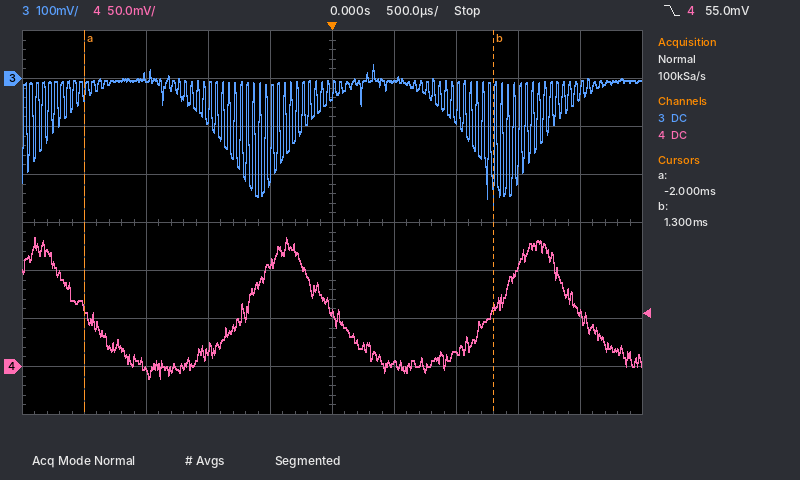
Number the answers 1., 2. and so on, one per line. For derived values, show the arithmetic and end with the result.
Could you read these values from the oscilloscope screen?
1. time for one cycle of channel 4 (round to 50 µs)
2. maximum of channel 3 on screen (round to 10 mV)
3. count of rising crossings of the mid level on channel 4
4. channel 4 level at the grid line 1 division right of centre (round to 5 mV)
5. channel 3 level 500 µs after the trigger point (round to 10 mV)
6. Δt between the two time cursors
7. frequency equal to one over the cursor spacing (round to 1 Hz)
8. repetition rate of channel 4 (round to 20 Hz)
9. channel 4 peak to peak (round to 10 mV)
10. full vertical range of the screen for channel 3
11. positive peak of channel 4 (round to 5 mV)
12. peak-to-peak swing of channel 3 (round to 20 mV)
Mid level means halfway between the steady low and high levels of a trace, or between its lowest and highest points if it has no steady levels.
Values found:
1. 2.00 ms
2. 30 mV
3. 2
4. 5 mV
5. -10 mV
6. 1.3 ms − (-2 ms) = 3.30 ms
7. 1 / 3.30 ms ≈ 303 Hz
8. 1 / 2.00 ms ≈ 500 Hz
9. 150 mV
10. 800 mV
11. 135 mV
12. 300 mV
